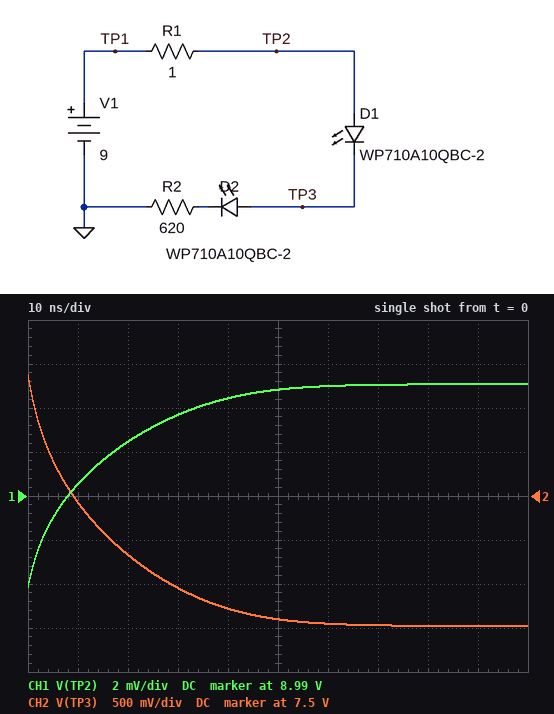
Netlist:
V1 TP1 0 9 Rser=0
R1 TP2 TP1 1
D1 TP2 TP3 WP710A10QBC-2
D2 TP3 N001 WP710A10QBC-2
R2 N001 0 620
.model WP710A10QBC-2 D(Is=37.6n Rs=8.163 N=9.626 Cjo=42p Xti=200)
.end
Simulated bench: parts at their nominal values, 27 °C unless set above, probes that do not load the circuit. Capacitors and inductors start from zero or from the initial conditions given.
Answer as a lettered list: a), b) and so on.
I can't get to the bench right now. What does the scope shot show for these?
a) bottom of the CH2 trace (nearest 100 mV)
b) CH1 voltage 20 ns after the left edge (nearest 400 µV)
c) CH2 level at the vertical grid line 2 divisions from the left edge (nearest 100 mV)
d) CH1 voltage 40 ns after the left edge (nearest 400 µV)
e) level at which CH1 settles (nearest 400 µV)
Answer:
a) 6.0 V
b) 8.9924 V
c) 6.8 V
d) 8.9944 V
e) 8.9952 V
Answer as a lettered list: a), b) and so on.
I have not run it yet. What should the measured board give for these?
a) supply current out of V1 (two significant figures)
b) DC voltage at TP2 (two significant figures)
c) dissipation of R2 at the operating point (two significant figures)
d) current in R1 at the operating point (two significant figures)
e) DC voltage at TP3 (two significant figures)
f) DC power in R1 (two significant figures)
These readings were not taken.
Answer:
a) 4.9 mA
b) 9.0 V
c) 15 mW
d) 4.9 mA
e) 6.0 V
f) 24 µW
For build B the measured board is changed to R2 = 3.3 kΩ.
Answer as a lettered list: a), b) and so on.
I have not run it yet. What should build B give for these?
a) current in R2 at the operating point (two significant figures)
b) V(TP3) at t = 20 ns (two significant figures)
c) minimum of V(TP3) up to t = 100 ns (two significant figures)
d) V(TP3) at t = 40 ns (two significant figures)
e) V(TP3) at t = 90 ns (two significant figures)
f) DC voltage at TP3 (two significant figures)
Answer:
a) 1.2 mA
b) 8.1 V
c) 6.9 V
d) 7.7 V
e) 7.0 V
f) 6.4 V
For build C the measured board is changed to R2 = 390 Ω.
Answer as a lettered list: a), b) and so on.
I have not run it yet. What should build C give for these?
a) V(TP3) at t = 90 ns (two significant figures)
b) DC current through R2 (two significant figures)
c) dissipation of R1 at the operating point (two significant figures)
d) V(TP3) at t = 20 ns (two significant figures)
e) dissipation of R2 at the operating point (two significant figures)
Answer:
a) 5.9 V
b) 7.2 mA
c) 52 µW
d) 6.4 V
e) 20 mW
